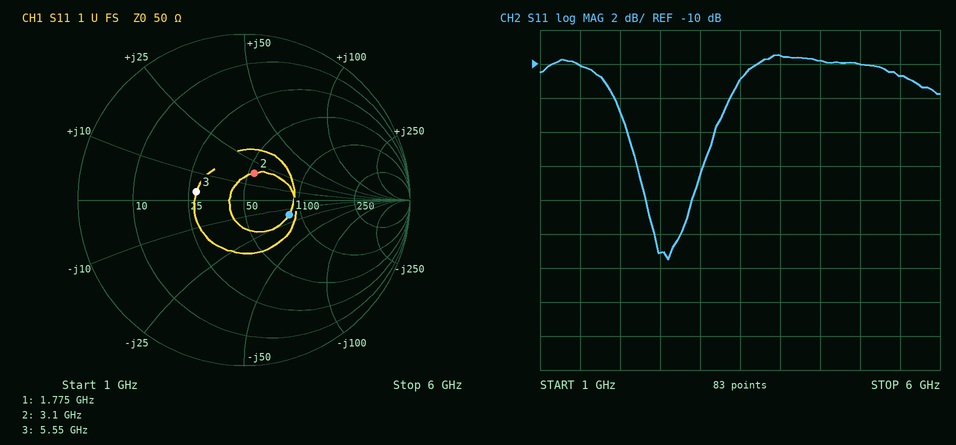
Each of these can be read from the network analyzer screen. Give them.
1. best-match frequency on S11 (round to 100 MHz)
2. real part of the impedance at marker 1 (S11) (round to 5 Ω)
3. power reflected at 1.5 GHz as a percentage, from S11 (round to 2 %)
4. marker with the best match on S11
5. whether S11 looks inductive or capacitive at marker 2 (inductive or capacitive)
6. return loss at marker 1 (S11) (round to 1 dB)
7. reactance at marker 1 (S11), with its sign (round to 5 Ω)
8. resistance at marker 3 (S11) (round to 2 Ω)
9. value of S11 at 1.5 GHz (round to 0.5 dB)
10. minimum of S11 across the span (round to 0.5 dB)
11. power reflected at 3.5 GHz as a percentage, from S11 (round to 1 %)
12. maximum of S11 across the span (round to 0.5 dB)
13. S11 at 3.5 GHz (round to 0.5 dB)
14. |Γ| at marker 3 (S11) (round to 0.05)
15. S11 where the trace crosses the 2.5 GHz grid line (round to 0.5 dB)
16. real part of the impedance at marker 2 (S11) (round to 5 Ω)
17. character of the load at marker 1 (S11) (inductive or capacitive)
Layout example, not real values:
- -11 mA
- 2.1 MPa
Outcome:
- 2.6 GHz
- 85 Ω
- 10 %
- marker 2
- inductive
- 11 dB
- -15 Ω
- 28 Ω
- -10.0 dB
- -21.5 dB
- 8 %
- -9.5 dB
- -11.0 dB
- 0.30
- -21.0 dB
- 55 Ω
- capacitive
